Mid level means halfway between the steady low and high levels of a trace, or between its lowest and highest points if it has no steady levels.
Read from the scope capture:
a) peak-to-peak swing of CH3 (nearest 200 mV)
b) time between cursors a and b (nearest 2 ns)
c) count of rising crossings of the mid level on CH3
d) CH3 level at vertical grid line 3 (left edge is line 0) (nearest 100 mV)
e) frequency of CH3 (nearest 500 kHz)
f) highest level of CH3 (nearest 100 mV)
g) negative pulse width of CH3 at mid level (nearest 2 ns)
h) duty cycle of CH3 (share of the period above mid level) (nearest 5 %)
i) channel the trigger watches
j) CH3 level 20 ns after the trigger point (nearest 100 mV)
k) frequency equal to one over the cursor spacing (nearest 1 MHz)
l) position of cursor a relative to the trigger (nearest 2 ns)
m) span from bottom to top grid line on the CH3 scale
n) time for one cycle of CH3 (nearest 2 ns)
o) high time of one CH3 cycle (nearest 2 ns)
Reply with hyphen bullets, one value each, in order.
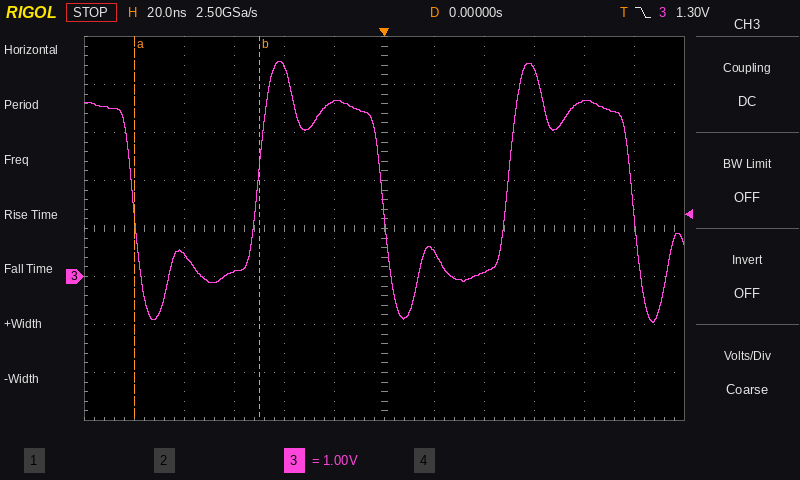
- 5.4 V
- 50 ns
- 2
- 100 mV
- 10.0 MHz
- 4.5 V
- 50 ns
- 50 %
- CH3
- 500 mV
- 20 MHz
- -100 ns
- 8 V
- 100 ns
- 50 ns
